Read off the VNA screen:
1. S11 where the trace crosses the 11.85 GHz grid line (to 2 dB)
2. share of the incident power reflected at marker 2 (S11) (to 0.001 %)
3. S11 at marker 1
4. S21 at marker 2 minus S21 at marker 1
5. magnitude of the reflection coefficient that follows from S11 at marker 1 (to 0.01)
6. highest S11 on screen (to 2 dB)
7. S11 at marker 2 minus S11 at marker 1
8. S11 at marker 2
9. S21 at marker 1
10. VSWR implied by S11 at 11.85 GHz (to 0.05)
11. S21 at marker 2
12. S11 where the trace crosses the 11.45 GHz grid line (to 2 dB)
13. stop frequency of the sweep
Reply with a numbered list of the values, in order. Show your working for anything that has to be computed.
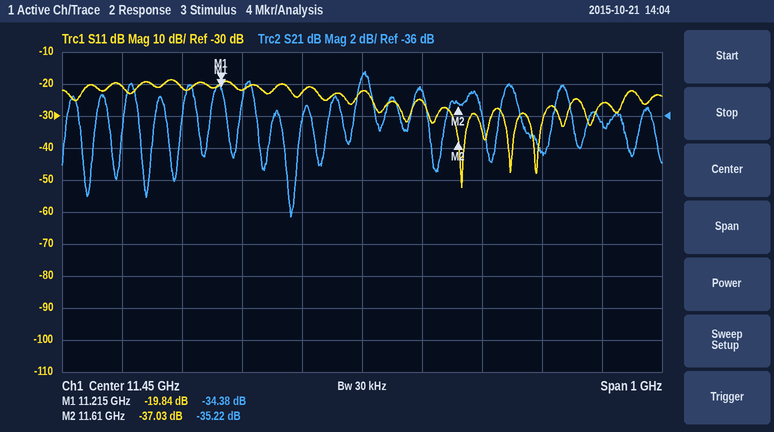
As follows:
1. -26 dB
2. 10^(-37.03/10) ≈ 0.020 %
3. -19.84 dB
4. -35.22 − (-34.38) = -0.84 dB
5. 10^(-19.84/20) ≈ 0.10
6. -18 dB
7. -37.03 − (-19.84) = -17.19 dB
8. -37.03 dB
9. -34.38 dB
10. |Γ| = 10^(-26/20) = 0.0501; VSWR = (1 + 0.0501)/(1 − 0.0501) ≈ 1.11, so 1.10 to the nearest 0.05
11. -35.22 dB
12. -22 dB
13. 11.95 GHz
